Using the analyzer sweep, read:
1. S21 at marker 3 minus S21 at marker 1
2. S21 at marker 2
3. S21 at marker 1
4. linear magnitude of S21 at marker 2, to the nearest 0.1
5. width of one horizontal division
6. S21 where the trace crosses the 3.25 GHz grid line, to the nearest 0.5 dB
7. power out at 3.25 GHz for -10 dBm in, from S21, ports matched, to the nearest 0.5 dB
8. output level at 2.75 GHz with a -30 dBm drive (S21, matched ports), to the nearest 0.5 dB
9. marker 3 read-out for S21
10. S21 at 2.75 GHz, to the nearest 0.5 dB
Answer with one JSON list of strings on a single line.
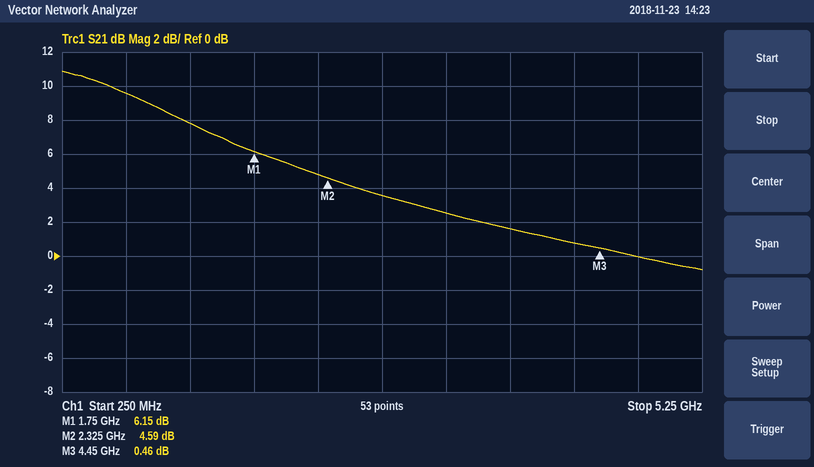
["-5.69 dB", "4.59 dB", "6.15 dB", "1.7", "500 MHz", "2.5 dB", "-7.5 dBm", "-26.5 dBm", "0.46 dB", "3.5 dB"]
